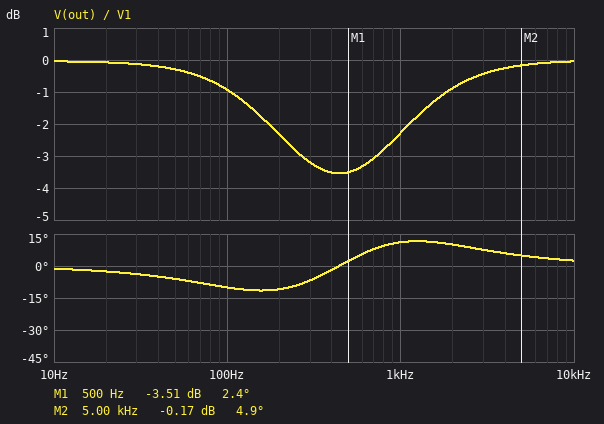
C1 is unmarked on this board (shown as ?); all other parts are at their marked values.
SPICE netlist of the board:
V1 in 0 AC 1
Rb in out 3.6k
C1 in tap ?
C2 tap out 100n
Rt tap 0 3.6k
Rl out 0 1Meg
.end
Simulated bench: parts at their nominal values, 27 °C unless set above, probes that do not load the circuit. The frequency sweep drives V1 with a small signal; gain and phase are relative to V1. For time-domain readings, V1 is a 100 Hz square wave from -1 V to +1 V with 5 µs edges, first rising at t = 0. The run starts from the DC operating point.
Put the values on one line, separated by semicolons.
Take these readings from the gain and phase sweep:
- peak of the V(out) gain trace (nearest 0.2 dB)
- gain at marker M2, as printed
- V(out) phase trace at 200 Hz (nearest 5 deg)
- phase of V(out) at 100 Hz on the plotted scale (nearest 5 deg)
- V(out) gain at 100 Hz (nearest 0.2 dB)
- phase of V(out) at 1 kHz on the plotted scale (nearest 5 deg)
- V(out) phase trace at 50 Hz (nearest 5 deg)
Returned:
0 dB; -0.17 dB; -10 deg; -10 deg; -1.0 dB; 10 deg; -5 deg
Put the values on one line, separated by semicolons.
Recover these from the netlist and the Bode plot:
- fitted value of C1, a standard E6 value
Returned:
100 nF
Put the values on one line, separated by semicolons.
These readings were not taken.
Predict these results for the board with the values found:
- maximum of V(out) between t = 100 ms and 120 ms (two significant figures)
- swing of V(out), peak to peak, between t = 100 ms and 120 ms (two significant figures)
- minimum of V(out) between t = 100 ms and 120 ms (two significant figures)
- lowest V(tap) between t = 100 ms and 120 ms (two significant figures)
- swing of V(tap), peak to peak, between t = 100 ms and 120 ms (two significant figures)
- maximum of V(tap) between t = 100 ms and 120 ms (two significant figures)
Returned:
990 mV; 2.0 V; -990 mV; -2.0 V; 4.0 V; 2.0 V
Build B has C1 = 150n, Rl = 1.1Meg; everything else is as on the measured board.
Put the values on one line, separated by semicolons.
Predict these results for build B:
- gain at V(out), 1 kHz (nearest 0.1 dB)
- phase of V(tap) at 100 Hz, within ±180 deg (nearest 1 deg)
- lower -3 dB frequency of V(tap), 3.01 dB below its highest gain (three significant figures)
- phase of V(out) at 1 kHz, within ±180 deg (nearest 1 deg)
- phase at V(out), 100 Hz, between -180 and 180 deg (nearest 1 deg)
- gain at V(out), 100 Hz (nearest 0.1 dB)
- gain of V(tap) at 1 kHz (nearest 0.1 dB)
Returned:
-1.5 dB; 57 deg; 226 Hz; 10 deg; -9 deg; -1.0 dB; -0.7 dB
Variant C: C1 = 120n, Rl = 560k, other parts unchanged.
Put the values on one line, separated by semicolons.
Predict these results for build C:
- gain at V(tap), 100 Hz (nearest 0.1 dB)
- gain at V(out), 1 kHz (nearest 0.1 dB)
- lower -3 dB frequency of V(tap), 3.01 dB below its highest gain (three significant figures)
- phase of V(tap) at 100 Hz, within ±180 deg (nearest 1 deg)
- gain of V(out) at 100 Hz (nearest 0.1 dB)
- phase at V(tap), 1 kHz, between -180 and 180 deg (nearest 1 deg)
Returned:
-7.5 dB; -1.9 dB; 285 Hz; 59 deg; -1.0 dB; 16 deg
